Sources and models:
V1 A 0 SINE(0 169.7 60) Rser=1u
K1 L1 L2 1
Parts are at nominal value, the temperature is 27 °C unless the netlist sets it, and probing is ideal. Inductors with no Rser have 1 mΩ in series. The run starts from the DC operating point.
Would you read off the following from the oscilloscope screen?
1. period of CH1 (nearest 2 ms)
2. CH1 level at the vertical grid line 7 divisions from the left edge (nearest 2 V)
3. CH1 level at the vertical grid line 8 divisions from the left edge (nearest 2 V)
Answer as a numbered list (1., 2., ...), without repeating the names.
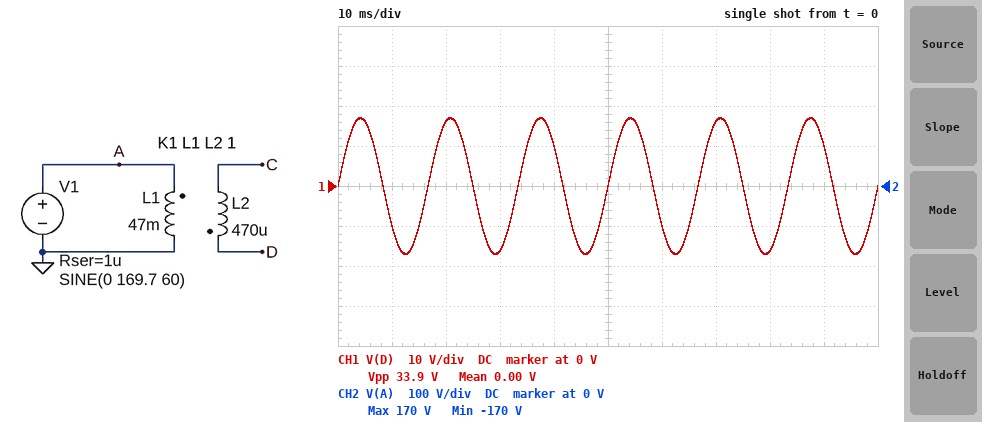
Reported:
1. 16 ms
2. 16 V
3. -16 V
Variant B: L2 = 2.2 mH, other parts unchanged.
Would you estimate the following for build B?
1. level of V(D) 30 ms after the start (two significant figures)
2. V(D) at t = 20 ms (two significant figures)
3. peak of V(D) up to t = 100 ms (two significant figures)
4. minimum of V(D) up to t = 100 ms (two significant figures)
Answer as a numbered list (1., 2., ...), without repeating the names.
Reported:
1. -35 V
2. 35 V
3. 37 V
4. -37 V
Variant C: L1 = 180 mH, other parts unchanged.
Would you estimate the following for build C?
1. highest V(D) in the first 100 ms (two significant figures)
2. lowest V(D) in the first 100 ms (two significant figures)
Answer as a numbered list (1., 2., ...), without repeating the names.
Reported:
1. 8.7 V
2. -8.7 V
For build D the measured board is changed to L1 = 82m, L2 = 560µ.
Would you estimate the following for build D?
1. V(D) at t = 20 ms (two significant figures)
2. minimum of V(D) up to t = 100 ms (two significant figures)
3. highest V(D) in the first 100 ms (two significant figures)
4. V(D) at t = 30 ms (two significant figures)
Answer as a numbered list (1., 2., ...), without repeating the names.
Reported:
1. 13 V
2. -14 V
3. 14 V
4. -13 V
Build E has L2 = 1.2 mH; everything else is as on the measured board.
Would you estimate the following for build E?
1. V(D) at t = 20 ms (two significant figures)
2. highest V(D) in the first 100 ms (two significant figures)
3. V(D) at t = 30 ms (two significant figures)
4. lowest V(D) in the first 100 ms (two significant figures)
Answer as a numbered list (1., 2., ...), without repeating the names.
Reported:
1. 26 V
2. 27 V
3. -26 V
4. -27 V
